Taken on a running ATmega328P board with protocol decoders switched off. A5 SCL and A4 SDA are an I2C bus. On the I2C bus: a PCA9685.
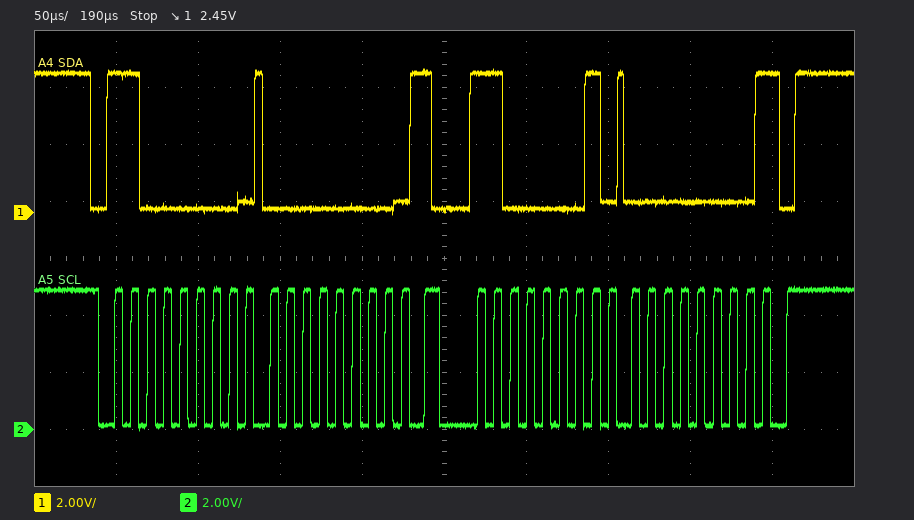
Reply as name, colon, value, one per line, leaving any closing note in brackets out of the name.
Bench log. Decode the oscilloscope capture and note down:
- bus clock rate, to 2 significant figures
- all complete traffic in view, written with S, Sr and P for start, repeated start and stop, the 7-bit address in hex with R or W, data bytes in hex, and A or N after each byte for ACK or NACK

bus clock rate, to 2 significant figures: 100 kHz
all complete traffic in view, written with S, Sr and P for start, repeated start and stop, the 7-bit address in hex with R or W, data bytes in hex, and A or N after each byte for ACK or NACK: S 60W A 00 A Sr 60R A 00 N P
